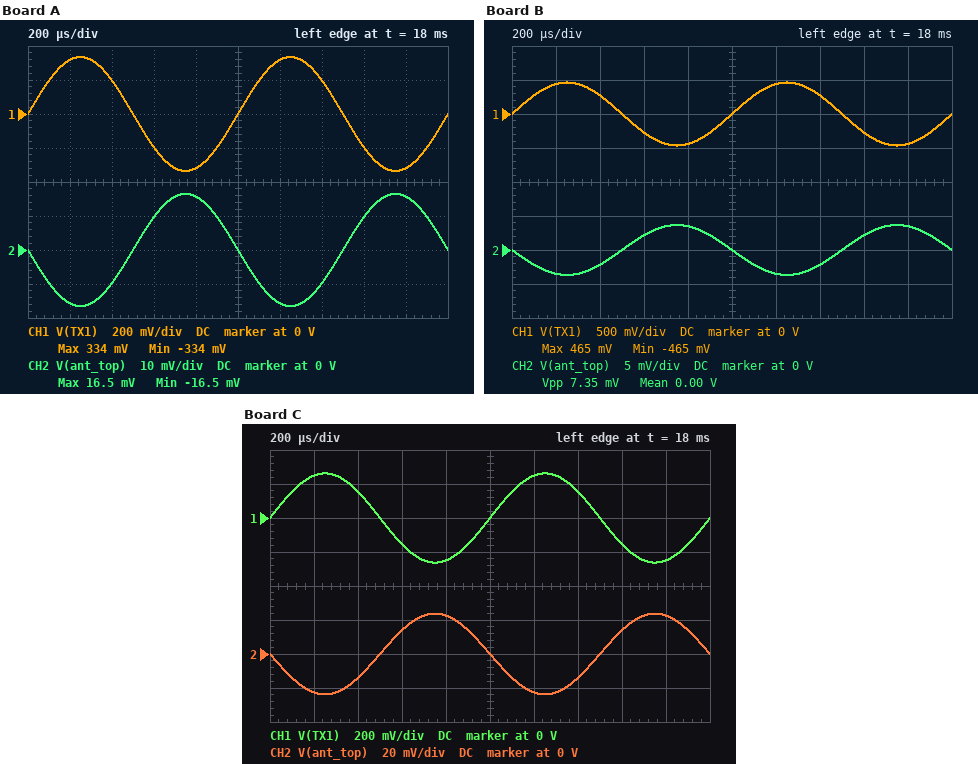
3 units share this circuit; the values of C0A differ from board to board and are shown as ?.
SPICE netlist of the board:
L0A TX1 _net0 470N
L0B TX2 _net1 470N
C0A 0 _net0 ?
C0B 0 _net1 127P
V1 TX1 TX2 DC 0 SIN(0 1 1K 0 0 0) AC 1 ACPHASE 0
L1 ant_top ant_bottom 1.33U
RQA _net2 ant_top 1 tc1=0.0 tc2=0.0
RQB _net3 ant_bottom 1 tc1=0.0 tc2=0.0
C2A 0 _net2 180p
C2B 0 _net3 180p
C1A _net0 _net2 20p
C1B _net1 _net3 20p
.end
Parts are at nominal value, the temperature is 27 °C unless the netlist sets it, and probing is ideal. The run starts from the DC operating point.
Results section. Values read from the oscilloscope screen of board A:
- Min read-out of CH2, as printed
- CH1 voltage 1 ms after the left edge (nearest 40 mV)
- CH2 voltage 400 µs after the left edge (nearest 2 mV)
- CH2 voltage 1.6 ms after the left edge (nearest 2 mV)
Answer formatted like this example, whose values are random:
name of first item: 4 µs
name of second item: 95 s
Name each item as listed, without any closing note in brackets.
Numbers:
Min read-out of CH2, as printed: -16.5 mV
CH1 voltage 1 ms after the left edge: 0 V
CH2 voltage 400 µs after the left edge: -10 mV
CH2 voltage 1.6 ms after the left edge: 10 mV
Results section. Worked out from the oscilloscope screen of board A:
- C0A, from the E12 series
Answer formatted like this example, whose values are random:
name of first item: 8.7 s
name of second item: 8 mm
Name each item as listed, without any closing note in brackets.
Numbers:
C0A, from the E12 series: 270 pF
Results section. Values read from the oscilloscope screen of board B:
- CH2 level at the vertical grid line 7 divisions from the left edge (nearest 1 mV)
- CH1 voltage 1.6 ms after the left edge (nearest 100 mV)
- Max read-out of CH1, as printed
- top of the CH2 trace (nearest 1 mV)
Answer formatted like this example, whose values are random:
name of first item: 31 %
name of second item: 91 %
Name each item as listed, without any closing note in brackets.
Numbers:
CH2 level at the vertical grid line 7 divisions from the left edge: -2 mV
CH1 voltage 1.6 ms after the left edge: -300 mV
Max read-out of CH1, as printed: 465 mV
top of the CH2 trace: 4 mV
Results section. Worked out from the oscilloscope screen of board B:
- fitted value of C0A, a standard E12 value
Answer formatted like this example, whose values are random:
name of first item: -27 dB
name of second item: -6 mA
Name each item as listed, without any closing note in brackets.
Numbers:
fitted value of C0A, a standard E12 value: 150 pF
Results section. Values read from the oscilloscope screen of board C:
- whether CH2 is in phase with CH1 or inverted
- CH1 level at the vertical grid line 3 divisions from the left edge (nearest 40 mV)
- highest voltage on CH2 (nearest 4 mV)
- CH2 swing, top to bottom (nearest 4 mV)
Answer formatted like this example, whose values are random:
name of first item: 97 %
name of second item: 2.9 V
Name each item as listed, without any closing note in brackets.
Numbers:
whether CH2 is in phase with CH1 or inverted: inverted
CH1 level at the vertical grid line 3 divisions from the left edge: -160 mV
highest voltage on CH2: 24 mV
CH2 swing, top to bottom: 48 mV
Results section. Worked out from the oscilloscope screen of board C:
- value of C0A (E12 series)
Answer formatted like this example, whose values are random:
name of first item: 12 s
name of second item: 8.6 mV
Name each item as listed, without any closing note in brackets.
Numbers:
value of C0A: 390 pF
